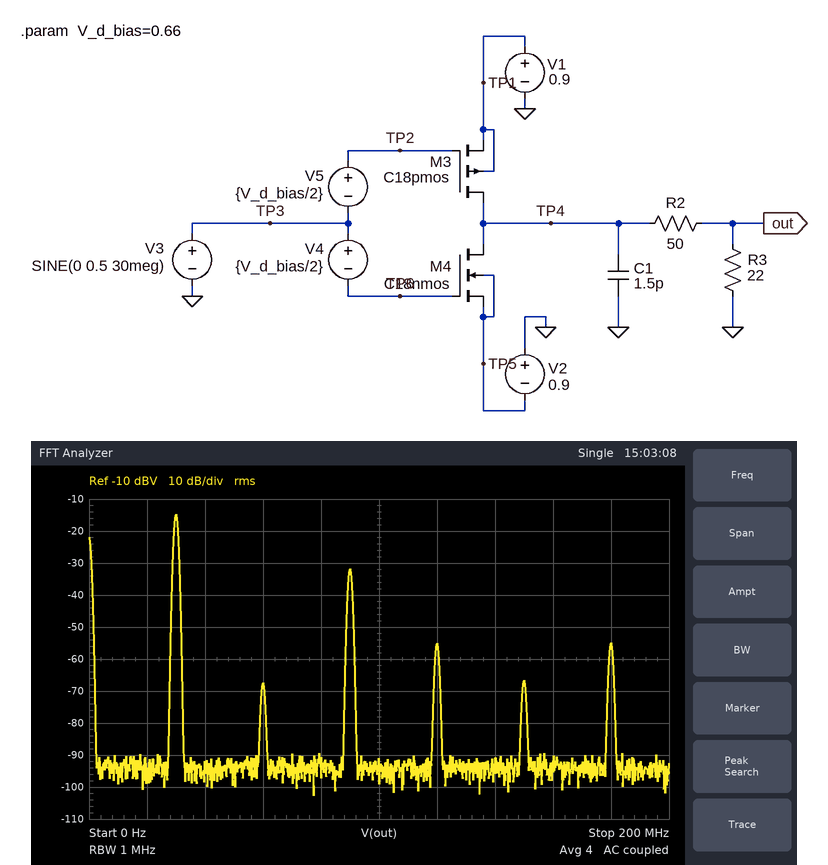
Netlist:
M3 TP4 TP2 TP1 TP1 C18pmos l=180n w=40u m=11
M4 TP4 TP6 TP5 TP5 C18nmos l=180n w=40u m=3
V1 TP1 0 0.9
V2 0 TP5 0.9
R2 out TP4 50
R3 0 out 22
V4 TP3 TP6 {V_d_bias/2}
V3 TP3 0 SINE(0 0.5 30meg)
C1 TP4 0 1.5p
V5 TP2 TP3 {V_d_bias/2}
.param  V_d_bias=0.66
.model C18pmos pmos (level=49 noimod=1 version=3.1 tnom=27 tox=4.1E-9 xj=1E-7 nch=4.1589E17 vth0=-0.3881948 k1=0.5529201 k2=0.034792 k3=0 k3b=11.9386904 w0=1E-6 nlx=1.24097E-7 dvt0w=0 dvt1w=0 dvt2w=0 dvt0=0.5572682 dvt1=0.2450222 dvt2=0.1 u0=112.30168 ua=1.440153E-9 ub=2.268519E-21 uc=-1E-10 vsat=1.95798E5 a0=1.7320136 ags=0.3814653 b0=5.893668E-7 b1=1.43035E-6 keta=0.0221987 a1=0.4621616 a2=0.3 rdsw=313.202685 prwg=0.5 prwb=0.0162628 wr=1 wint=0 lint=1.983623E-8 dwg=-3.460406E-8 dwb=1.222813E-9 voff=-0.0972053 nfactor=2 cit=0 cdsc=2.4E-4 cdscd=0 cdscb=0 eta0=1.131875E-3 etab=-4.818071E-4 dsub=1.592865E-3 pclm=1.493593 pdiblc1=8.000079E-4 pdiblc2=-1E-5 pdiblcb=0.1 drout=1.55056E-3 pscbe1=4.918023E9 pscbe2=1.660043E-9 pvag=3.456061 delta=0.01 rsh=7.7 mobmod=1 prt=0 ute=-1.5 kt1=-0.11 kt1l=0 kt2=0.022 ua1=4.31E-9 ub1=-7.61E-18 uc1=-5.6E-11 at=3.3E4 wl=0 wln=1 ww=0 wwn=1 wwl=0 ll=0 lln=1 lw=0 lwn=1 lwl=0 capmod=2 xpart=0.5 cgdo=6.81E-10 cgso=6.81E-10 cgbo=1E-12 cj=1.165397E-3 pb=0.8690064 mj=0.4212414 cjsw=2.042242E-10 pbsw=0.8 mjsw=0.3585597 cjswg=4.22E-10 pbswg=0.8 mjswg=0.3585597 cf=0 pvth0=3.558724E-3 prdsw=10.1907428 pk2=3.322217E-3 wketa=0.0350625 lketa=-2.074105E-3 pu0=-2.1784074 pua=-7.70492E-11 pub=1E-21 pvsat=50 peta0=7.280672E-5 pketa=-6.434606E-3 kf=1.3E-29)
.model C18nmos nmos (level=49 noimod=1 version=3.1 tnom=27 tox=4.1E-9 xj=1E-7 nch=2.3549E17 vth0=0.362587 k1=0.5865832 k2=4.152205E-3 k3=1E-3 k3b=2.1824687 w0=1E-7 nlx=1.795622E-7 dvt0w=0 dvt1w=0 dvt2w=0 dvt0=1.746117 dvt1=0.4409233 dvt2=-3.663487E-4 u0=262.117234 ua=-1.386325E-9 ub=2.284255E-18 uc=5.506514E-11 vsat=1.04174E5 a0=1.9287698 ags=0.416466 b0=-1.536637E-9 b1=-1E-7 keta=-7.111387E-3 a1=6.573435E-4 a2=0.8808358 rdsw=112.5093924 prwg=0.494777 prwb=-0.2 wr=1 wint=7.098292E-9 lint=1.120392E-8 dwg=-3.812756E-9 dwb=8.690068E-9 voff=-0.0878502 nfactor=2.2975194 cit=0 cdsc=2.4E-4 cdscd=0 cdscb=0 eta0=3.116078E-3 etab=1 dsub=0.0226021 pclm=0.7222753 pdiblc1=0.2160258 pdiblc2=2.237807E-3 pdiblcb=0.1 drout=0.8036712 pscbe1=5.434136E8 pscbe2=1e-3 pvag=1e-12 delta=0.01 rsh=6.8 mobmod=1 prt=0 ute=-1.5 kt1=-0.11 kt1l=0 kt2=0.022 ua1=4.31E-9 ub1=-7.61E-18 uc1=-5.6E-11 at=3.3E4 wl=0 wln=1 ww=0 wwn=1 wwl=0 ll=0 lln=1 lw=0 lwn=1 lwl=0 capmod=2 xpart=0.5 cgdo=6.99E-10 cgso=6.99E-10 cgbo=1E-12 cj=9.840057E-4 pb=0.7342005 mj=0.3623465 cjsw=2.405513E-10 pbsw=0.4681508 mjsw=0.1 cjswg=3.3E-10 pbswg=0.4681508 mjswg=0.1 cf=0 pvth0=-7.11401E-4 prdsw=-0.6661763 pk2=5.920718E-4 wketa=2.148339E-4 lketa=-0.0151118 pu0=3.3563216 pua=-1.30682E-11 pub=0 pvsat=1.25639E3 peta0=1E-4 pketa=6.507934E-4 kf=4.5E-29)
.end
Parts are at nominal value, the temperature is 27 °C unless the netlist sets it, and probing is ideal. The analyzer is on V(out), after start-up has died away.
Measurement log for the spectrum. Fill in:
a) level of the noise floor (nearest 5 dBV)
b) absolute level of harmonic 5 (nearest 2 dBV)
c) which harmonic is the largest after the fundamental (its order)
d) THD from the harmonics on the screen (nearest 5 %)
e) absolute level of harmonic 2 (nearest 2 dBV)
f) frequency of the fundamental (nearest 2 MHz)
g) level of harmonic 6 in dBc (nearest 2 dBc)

-95 dBV
-66 dBV
3
15 %
-68 dBV
30 MHz
-40 dBc
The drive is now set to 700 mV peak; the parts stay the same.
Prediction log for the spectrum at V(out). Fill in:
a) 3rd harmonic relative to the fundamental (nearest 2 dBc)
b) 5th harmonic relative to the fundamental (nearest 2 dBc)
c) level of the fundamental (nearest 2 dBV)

-14 dBc
-26 dBc
-14 dBV
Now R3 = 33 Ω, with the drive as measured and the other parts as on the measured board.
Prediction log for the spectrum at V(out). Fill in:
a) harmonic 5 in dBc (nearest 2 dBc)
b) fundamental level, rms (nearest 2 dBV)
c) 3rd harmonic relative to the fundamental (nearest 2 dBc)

-36 dBc
-12 dBV
-16 dBc
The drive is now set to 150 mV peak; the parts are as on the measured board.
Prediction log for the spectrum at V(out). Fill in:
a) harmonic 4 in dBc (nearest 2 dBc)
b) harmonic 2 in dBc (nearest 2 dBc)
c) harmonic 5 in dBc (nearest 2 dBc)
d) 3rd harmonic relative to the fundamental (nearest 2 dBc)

-56 dBc
-30 dBc
-50 dBc
-34 dBc
